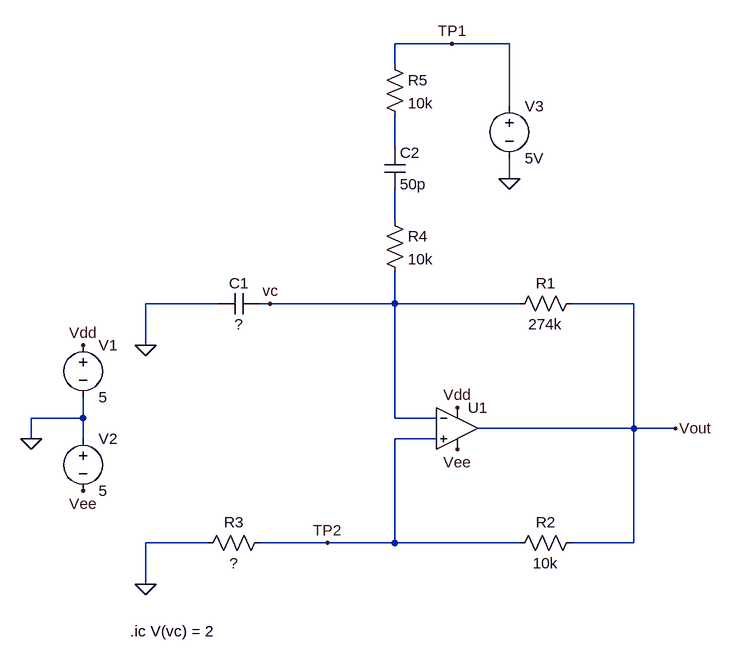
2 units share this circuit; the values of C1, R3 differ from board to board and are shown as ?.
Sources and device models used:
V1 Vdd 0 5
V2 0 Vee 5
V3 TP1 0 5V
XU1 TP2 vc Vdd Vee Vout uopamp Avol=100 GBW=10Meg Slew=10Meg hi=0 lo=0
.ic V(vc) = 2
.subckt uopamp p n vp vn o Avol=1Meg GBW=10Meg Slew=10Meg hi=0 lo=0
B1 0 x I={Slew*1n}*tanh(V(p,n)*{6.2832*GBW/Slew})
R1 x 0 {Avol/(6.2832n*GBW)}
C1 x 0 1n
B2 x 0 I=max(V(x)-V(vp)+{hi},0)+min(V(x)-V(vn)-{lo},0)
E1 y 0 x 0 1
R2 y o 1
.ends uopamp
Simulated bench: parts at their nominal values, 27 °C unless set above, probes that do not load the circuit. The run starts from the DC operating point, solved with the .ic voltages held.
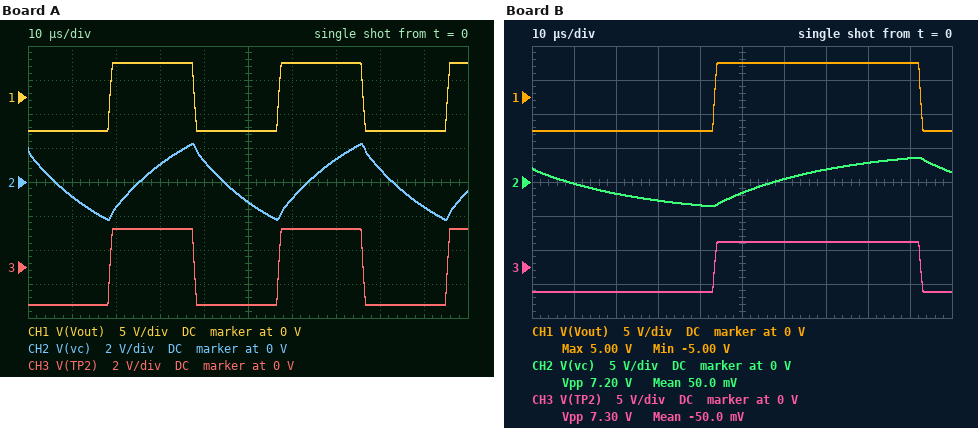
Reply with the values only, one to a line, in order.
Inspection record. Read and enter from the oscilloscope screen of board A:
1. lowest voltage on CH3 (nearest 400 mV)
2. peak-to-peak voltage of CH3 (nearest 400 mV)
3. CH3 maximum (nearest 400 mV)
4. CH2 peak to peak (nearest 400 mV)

-2.4 V
4.4 V
2.4 V
4.4 V
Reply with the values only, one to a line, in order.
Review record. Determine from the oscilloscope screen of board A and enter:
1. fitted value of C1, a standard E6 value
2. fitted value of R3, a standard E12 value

22 pF
8.2 kΩ
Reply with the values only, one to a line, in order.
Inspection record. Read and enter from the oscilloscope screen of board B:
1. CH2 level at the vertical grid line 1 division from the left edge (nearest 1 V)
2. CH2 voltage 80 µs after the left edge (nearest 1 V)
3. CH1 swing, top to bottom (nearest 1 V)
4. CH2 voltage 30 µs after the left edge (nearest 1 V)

0 V
3 V
10 V
-3 V
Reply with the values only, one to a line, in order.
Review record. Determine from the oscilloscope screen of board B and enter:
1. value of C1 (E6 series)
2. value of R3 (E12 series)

47 pF
27 kΩ
